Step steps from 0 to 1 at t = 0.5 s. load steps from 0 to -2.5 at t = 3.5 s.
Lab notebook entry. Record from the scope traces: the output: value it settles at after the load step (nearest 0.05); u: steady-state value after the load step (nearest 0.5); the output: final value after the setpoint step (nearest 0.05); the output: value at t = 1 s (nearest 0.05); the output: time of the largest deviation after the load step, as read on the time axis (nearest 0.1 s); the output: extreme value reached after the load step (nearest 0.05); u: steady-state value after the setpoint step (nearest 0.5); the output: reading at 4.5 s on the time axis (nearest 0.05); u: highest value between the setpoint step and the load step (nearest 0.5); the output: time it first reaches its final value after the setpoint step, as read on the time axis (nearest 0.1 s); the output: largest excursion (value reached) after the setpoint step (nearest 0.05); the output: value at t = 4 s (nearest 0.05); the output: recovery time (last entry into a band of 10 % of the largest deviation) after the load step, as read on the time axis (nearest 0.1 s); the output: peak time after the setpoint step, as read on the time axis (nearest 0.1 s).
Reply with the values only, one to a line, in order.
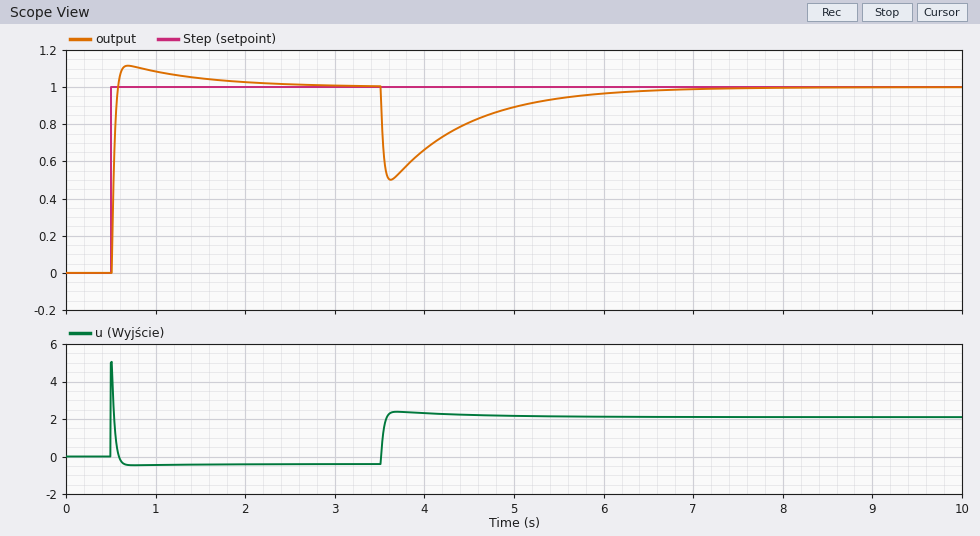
1.00
2.0
1.00
1.10
3.6 s
0.50
-0.5
0.80
5.0
0.6 s
1.10
0.65
5.7 s
0.7 s
